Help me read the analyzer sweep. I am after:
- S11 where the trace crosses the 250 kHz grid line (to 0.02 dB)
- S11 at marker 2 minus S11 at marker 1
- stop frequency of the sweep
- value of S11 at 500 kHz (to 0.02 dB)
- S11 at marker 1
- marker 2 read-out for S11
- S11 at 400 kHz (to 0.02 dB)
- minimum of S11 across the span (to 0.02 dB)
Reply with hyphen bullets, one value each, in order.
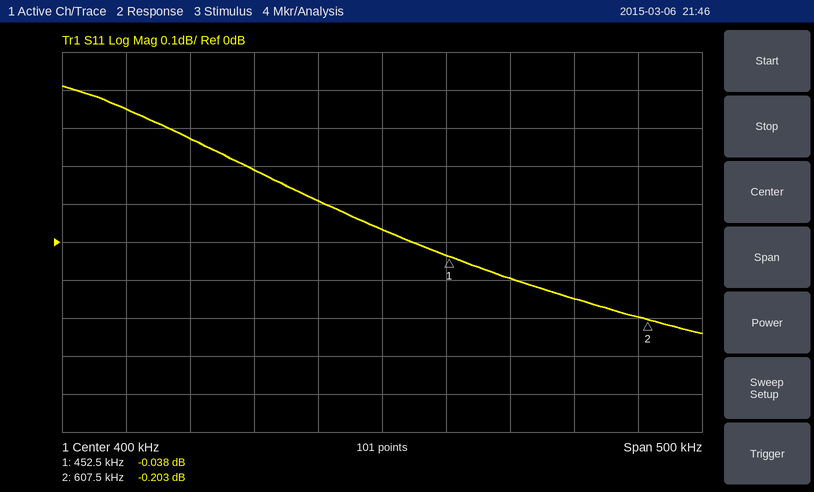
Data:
- 0.28 dB
- -0.165 dB
- 650 kHz
- -0.10 dB
- -0.038 dB
- -0.203 dB
- 0.04 dB
- -0.24 dB
